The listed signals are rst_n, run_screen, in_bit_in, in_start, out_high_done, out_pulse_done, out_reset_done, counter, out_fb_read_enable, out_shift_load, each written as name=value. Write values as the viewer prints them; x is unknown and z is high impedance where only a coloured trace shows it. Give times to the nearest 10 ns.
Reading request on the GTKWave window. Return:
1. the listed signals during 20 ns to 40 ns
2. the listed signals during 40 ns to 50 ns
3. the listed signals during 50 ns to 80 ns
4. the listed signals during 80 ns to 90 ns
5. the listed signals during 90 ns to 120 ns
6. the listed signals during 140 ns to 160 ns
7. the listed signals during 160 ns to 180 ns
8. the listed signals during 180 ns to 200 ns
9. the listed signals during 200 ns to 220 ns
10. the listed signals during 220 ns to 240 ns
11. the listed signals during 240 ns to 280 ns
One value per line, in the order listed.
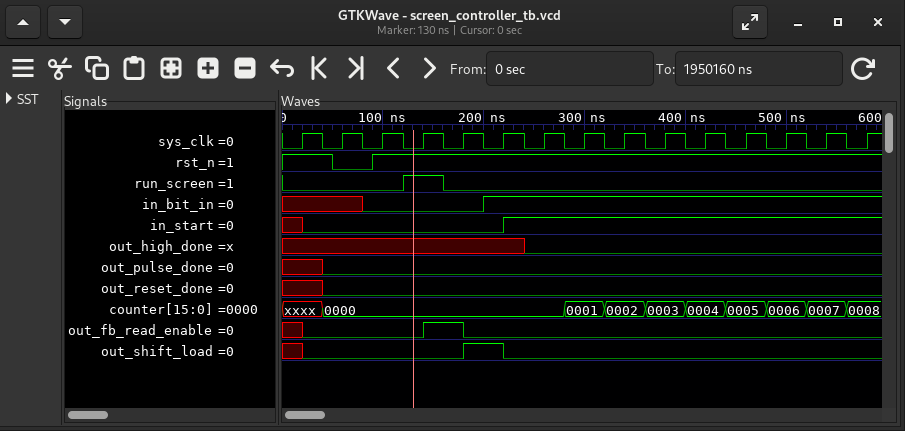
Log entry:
rst_n=1, run_screen=0, in_bit_in=x, in_start=0, out_high_done=x, out_pulse_done=x, out_reset_done=x, counter=xxxx, out_fb_read_enable=0, out_shift_load=0
rst_n=1, run_screen=0, in_bit_in=x, in_start=0, out_high_done=x, out_pulse_done=0, out_reset_done=0, counter=0000, out_fb_read_enable=0, out_shift_load=0
rst_n=0, run_screen=0, in_bit_in=x, in_start=0, out_high_done=x, out_pulse_done=0, out_reset_done=0, counter=0000, out_fb_read_enable=0, out_shift_load=0
rst_n=0, run_screen=0, in_bit_in=0, in_start=0, out_high_done=x, out_pulse_done=0, out_reset_done=0, counter=0000, out_fb_read_enable=0, out_shift_load=0
rst_n=1, run_screen=0, in_bit_in=0, in_start=0, out_high_done=x, out_pulse_done=0, out_reset_done=0, counter=0000, out_fb_read_enable=0, out_shift_load=0
rst_n=1, run_screen=1, in_bit_in=0, in_start=0, out_high_done=x, out_pulse_done=0, out_reset_done=0, counter=0000, out_fb_read_enable=1, out_shift_load=0
rst_n=1, run_screen=0, in_bit_in=0, in_start=0, out_high_done=x, out_pulse_done=0, out_reset_done=0, counter=0000, out_fb_read_enable=1, out_shift_load=0
rst_n=1, run_screen=0, in_bit_in=0, in_start=0, out_high_done=x, out_pulse_done=0, out_reset_done=0, counter=0000, out_fb_read_enable=0, out_shift_load=1
rst_n=1, run_screen=0, in_bit_in=1, in_start=0, out_high_done=x, out_pulse_done=0, out_reset_done=0, counter=0000, out_fb_read_enable=0, out_shift_load=1
rst_n=1, run_screen=0, in_bit_in=1, in_start=1, out_high_done=x, out_pulse_done=0, out_reset_done=0, counter=0000, out_fb_read_enable=0, out_shift_load=0
rst_n=1, run_screen=0, in_bit_in=1, in_start=1, out_high_done=0, out_pulse_done=0, out_reset_done=0, counter=0000, out_fb_read_enable=0, out_shift_load=0
